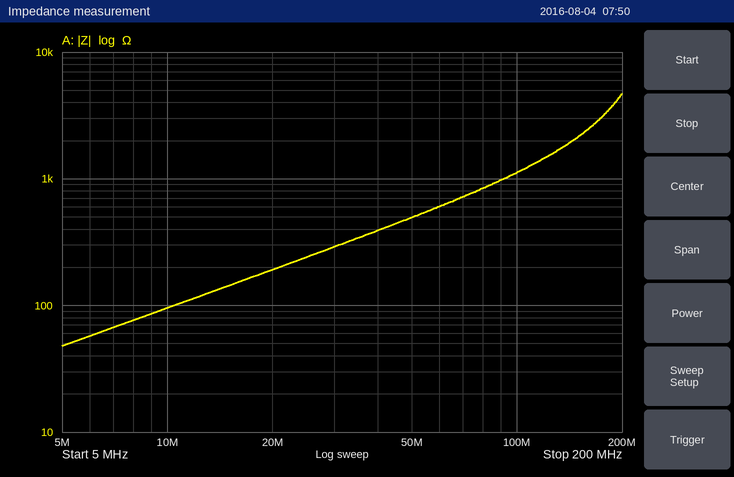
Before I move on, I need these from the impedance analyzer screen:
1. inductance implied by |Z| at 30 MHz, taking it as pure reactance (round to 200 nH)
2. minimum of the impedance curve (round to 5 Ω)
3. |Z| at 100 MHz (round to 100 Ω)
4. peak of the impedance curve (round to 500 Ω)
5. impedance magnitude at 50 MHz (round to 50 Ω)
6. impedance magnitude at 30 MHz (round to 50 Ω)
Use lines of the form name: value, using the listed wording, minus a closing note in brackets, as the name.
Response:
inductance implied by |Z| at 30 MHz, taking it as pure reactance: 1.6 µH
minimum of the impedance curve: 50 Ω
|Z| at 100 MHz: 1.1 kΩ
peak of the impedance curve: 4.5 kΩ
impedance magnitude at 50 MHz: 500 Ω
impedance magnitude at 30 MHz: 300 Ω
